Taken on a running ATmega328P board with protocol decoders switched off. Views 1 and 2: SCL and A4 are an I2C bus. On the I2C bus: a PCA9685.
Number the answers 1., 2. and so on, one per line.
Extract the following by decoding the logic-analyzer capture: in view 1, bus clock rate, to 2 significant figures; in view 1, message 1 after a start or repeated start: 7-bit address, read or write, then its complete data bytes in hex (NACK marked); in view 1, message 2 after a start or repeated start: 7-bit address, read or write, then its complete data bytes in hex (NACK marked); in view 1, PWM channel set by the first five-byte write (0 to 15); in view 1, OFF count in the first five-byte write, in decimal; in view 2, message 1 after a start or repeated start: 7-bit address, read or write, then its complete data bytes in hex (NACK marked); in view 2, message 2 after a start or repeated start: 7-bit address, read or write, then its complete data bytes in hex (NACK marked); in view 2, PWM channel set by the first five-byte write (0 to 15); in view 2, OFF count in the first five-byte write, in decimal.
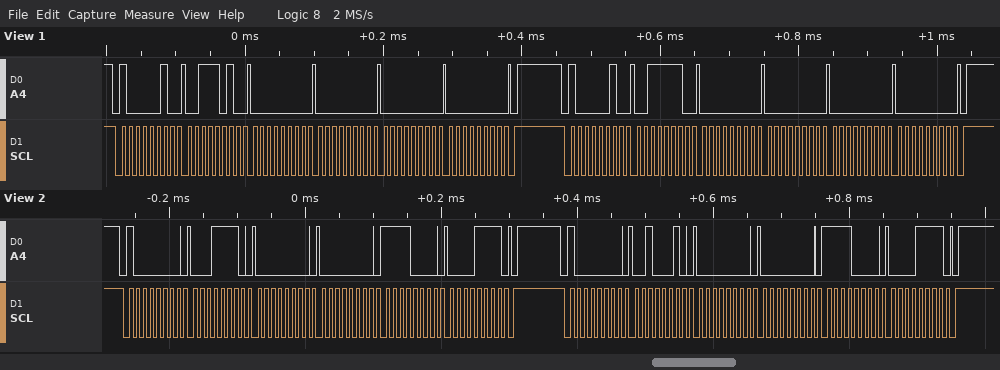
1. 100 kHz
2. 0x41 write: 3A 00 00 00 00
3. 0x41 write: 3E 00 00 00 00
4. 13
5. 0
6. 0x40 write: 1E 00 00 F0 0F
7. 0x40 write: 22 00 00 F0 0F
8. 6
9. 4080
